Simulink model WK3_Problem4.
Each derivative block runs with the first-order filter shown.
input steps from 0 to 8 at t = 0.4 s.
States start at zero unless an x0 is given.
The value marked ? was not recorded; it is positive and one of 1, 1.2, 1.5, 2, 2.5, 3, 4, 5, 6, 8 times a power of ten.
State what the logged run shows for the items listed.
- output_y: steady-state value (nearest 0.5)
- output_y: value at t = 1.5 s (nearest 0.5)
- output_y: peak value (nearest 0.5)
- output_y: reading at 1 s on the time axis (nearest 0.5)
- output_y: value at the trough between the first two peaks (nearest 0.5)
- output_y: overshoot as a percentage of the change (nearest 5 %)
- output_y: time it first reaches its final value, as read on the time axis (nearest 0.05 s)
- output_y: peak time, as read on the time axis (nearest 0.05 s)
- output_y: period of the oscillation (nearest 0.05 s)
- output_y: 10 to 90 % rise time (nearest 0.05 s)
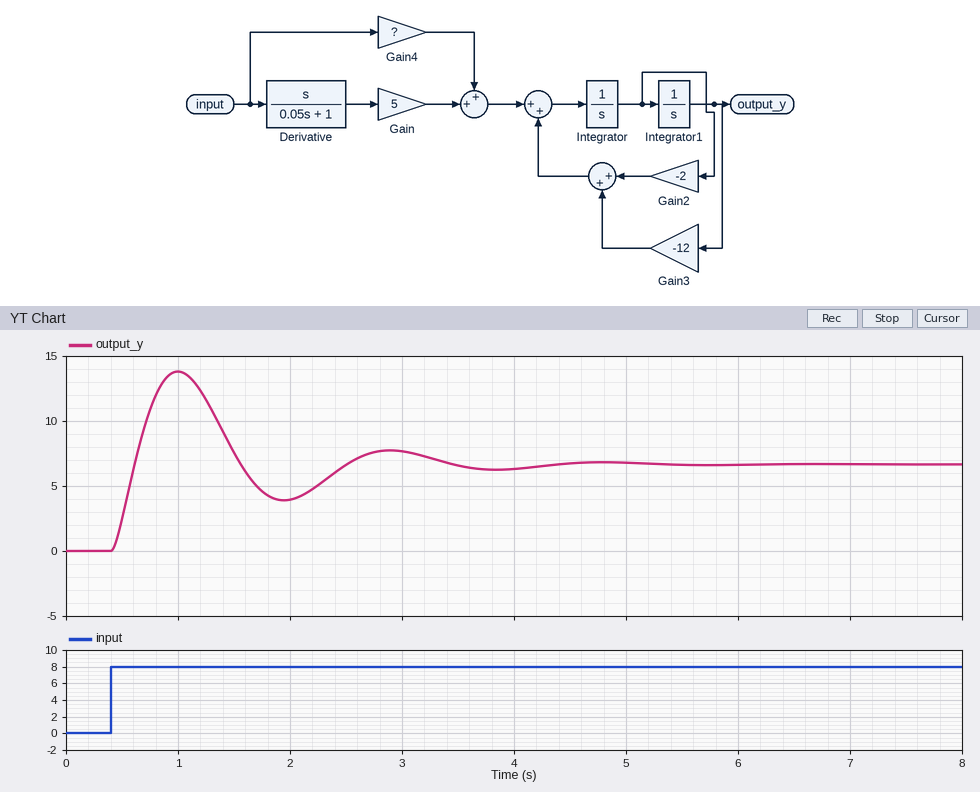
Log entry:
6.5
7.5
14.0
14.0
4.0
105 %
0.60 s
1.00 s
1.90 s
0.15 s
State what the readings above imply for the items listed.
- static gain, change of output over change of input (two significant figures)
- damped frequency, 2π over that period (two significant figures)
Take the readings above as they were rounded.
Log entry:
0.81
3.3 rad/s
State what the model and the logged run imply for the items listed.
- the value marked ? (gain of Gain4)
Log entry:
10
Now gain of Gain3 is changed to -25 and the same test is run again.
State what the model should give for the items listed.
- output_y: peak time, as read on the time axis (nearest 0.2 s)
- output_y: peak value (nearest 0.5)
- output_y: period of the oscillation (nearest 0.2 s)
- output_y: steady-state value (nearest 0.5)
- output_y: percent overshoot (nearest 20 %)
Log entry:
0.8 s
9.0
1.2 s
3.0
180 %
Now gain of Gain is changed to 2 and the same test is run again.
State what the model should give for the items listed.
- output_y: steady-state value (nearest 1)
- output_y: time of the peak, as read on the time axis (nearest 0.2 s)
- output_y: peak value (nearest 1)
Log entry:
7
1.2 s
10
